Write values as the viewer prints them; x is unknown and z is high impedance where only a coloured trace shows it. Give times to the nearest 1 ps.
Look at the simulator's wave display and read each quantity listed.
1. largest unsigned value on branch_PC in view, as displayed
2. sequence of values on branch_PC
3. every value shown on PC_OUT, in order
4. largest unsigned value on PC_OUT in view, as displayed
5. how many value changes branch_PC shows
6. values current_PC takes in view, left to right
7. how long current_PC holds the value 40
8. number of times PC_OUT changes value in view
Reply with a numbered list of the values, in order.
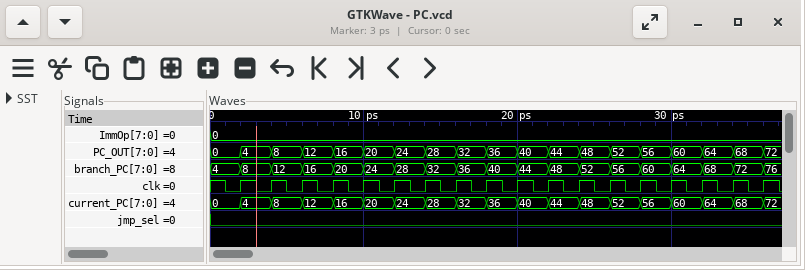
1. 76
2. 4, 8, 12, 16, 20, 24, 28, 32, 36, 40, 44, 48, 52, 56, 60, 64, 68, 72, 76
3. 0, 4, 8, 12, 16, 20, 24, 28, 32, 36, 40, 44, 48, 52, 56, 60, 64, 68, 72
4. 72
5. 18
6. 0, 4, 8, 12, 16, 20, 24, 28, 32, 36, 40, 44, 48, 52, 56, 60, 64, 68, 72
7. 2 ps
8. 18
